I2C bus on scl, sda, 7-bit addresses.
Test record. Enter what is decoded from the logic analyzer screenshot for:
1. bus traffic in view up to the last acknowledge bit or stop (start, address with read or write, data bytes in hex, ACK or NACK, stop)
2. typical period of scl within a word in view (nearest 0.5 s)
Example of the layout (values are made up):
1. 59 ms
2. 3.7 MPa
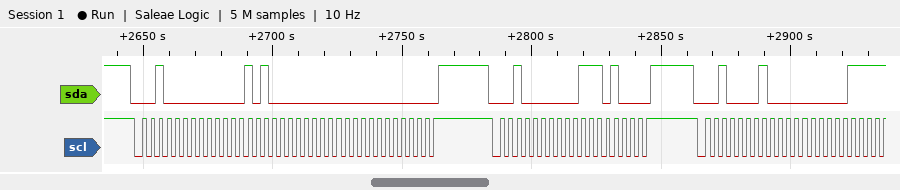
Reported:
1. start, address 10 write ACK, 0A ACK, 00 ACK, 00 ACK, stop, start, address 10 write ACK, 74 ACK, stop, start, address 10 read ACK, 00 ACK
2. 3 s
